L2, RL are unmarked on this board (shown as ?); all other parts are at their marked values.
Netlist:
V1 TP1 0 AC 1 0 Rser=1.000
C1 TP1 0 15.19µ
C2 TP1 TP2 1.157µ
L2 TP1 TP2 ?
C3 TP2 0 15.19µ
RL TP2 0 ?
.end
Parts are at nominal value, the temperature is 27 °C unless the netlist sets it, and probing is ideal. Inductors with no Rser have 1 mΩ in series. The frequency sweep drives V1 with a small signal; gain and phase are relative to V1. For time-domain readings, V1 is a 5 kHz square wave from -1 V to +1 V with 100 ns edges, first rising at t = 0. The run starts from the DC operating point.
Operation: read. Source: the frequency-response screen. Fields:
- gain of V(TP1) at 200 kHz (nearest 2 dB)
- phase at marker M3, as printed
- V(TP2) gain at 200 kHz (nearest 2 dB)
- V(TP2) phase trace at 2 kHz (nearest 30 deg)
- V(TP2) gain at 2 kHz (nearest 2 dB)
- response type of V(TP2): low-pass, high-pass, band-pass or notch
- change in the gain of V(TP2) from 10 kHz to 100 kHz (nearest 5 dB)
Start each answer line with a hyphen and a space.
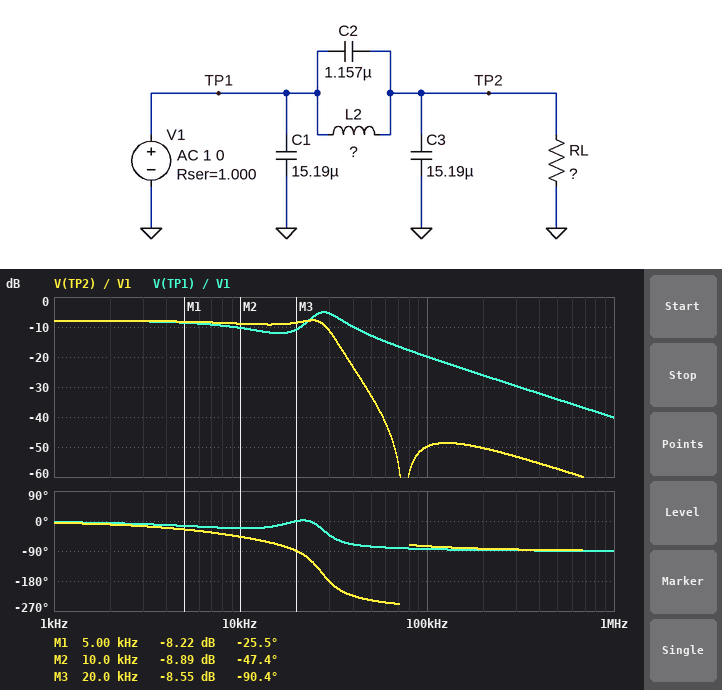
- -26 dB
- -90.4 deg
- -50 dB
- 0 deg
- -8 dB
- low-pass
- -40 dB
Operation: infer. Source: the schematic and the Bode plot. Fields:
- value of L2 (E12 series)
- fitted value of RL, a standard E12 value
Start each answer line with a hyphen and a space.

- 3.9 µH
- 0.68 Ω
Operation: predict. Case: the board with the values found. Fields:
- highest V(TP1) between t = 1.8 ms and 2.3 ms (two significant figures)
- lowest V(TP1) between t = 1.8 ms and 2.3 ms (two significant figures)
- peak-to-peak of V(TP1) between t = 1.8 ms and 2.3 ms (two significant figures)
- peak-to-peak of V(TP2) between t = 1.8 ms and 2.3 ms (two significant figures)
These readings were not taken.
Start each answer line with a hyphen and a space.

- 460 mV
- -460 mV
- 920 mV
- 910 mV
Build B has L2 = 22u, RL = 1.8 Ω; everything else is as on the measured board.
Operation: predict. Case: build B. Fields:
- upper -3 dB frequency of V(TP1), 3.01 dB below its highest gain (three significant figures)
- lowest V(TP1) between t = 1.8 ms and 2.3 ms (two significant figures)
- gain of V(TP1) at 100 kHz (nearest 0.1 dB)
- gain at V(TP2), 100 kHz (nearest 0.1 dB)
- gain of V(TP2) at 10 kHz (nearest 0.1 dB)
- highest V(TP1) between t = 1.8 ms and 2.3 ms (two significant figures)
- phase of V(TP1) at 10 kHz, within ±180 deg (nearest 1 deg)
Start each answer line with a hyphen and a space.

- 18.5 kHz
- -690 mV
- -20.2 dB
- -44.0 dB
- -3.8 dB
- 690 mV
- 1 deg
